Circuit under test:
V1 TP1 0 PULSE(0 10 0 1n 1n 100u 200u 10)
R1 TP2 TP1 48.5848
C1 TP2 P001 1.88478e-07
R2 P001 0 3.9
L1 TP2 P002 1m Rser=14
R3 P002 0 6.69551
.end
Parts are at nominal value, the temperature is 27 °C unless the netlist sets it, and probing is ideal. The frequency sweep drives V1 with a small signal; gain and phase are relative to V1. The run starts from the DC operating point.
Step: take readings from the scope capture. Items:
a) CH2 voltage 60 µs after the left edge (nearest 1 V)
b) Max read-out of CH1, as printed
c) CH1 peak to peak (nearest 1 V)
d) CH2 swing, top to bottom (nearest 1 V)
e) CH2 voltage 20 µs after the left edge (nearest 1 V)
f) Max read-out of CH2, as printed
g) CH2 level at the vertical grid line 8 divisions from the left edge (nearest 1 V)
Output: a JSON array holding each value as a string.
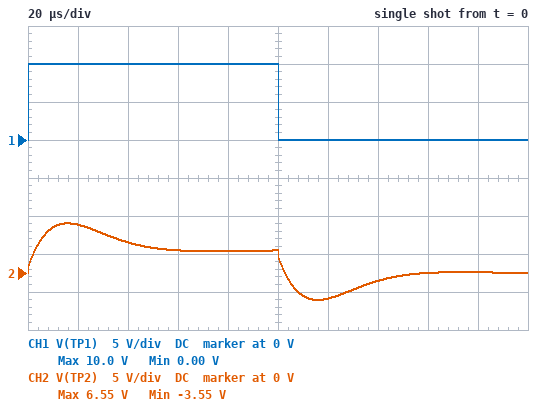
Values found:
["3 V", "10.0 V", "10 V", "10 V", "6 V", "6.55 V", "0 V"]
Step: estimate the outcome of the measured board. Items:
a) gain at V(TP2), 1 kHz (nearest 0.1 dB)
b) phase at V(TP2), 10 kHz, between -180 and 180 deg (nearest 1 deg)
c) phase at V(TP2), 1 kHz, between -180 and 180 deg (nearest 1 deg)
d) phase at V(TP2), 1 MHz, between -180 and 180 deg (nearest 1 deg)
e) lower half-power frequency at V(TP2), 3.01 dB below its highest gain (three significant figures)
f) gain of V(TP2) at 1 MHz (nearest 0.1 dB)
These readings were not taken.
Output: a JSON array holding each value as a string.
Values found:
["-10.1 dB", "6 deg", "11 deg", "-11 deg", "5.91 kHz", "-22.4 dB"]
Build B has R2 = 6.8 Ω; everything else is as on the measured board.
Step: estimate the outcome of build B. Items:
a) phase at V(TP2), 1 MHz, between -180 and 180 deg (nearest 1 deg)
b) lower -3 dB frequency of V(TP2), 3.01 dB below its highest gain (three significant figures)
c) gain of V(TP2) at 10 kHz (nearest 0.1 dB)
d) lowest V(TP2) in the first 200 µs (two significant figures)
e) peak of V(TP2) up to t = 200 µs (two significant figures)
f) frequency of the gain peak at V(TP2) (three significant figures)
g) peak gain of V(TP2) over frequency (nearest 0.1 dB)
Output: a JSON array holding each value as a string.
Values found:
["-6 deg", "5.72 kHz", "-2.2 dB", "-3.4 V", "6.4 V", "12.6 kHz", "-1.8 dB"]
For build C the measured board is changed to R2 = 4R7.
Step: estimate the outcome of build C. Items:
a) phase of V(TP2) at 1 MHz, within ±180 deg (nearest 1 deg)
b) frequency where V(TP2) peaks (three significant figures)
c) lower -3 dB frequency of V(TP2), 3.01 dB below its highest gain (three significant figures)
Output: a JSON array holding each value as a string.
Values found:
["-9 deg", "12.8 kHz", "5.86 kHz"]
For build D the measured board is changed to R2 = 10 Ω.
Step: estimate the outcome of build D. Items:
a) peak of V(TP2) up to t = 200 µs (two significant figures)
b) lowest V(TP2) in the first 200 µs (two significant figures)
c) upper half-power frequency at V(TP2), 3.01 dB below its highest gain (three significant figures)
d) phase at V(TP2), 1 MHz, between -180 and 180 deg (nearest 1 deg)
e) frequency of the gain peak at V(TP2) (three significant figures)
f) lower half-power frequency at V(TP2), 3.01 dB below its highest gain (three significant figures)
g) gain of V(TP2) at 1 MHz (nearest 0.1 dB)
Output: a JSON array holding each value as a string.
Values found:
["6.3 V", "-3.3 V", "25.5 kHz", "-4 deg", "12.3 kHz", "5.53 kHz", "-15.3 dB"]
